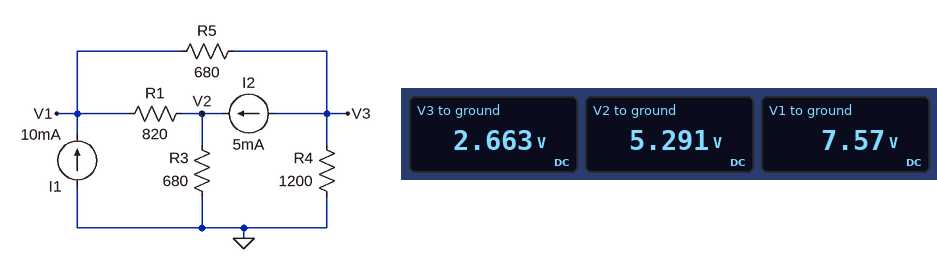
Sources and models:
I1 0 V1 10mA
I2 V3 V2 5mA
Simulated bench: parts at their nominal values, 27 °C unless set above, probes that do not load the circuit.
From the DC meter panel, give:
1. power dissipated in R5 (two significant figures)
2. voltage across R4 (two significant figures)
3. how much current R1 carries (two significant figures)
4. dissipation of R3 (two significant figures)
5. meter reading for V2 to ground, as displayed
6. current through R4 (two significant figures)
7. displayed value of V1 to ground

35 mW
2.7 V
2.8 mA
41 mW
5.291 V
2.2 mA
7.57 V
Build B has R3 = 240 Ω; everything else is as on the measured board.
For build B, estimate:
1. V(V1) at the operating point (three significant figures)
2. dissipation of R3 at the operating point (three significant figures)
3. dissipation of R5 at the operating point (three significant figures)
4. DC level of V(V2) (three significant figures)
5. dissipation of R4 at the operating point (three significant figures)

5.38 V
19.2 mW
24.9 mW
2.15 V
1.33 mW
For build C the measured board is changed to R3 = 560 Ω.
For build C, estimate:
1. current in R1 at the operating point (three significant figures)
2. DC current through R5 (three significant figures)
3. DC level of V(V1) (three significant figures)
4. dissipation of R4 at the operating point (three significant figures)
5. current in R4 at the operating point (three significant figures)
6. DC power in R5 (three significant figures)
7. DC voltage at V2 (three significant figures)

3.07 mA
6.93 mA
7.03 V
4.48 mW
1.93 mA
32.7 mW
4.52 V
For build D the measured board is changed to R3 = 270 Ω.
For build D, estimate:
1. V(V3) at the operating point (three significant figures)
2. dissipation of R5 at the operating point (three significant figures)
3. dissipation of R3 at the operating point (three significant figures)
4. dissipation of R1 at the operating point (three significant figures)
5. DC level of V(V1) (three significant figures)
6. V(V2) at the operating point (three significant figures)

1.37 V
25.7 mW
21.2 mW
12.2 mW
5.55 V
2.39 V
